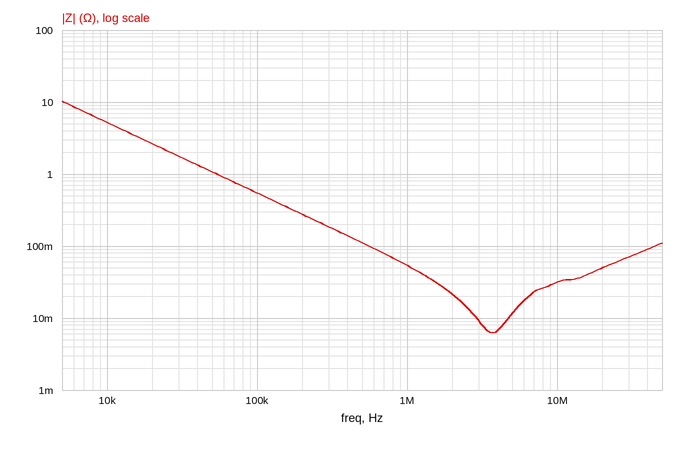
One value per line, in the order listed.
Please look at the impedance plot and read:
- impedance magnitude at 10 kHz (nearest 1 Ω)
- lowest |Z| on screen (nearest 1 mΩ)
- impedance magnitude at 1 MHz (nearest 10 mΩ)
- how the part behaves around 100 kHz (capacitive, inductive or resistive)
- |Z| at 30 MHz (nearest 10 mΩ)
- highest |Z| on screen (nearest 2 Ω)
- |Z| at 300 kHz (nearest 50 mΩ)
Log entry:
5 Ω
6 mΩ
50 mΩ
capacitive
70 mΩ
10 Ω
200 mΩ
